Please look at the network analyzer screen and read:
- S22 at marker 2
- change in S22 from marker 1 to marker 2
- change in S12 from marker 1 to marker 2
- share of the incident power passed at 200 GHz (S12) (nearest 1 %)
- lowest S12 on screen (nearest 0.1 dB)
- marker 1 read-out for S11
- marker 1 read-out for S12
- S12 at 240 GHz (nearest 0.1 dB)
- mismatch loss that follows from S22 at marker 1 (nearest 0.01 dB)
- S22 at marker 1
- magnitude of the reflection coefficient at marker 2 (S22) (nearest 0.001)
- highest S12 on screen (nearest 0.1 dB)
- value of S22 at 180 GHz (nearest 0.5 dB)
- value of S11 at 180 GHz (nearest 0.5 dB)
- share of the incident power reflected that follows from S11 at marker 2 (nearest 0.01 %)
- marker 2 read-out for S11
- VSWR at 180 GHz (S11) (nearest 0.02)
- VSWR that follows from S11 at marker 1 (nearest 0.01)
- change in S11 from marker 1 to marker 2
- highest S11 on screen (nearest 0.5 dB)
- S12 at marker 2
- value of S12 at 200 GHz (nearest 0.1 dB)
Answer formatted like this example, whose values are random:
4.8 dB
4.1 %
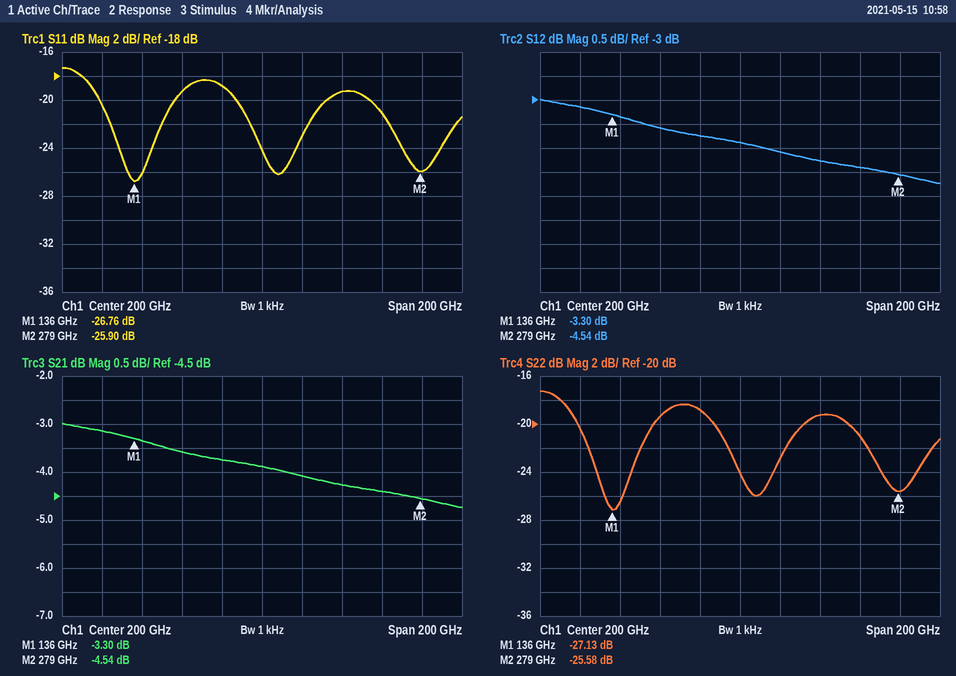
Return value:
-25.58 dB
1.55 dB
-1.24 dB
41 %
-4.7 dB
-26.76 dB
-3.30 dB
-4.3 dB
0.01 dB
-27.13 dB
0.053
-3.0 dB
-19.0 dB
-19.0 dB
0.26 %
-25.90 dB
1.26
1.10
0.86 dB
-17.5 dB
-4.54 dB
-3.9 dB
